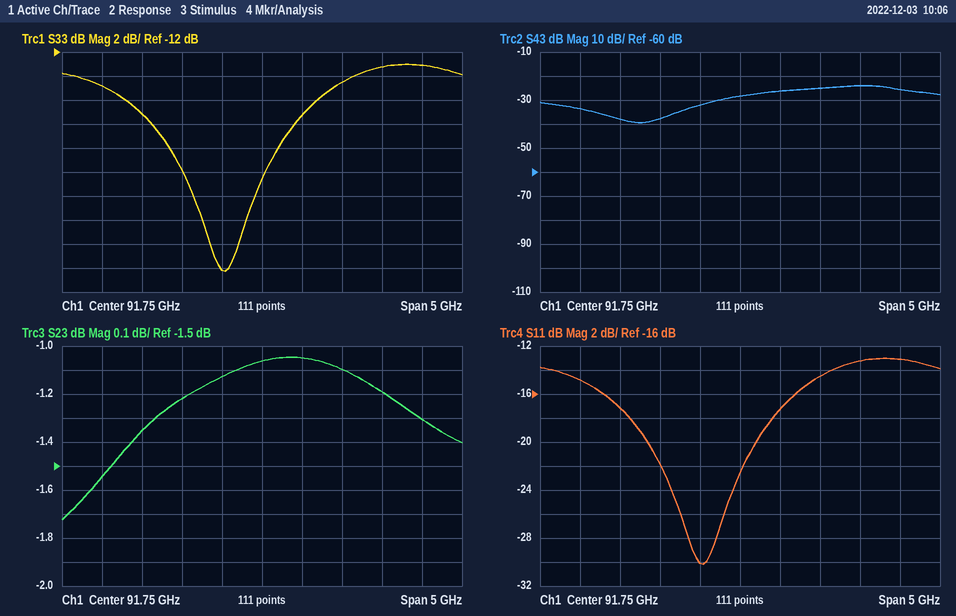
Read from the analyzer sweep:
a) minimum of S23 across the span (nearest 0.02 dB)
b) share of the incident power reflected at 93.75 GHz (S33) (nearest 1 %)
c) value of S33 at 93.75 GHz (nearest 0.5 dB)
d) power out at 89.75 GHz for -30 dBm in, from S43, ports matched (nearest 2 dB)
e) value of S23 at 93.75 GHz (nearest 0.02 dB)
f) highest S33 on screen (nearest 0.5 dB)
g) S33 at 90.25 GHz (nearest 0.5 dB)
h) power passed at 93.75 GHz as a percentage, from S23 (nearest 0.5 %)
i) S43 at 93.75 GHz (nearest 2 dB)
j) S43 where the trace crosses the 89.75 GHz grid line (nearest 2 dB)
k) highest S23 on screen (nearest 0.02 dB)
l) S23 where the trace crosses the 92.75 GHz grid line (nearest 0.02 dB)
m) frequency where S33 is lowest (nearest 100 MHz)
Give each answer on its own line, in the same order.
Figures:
-1.72 dB
5 %
-13.0 dB
-64 dBm
-1.30 dB
-13.0 dB
-17.0 dB
74.0 %
-26 dB
-34 dB
-1.04 dB
-1.10 dB
91.3 GHz
